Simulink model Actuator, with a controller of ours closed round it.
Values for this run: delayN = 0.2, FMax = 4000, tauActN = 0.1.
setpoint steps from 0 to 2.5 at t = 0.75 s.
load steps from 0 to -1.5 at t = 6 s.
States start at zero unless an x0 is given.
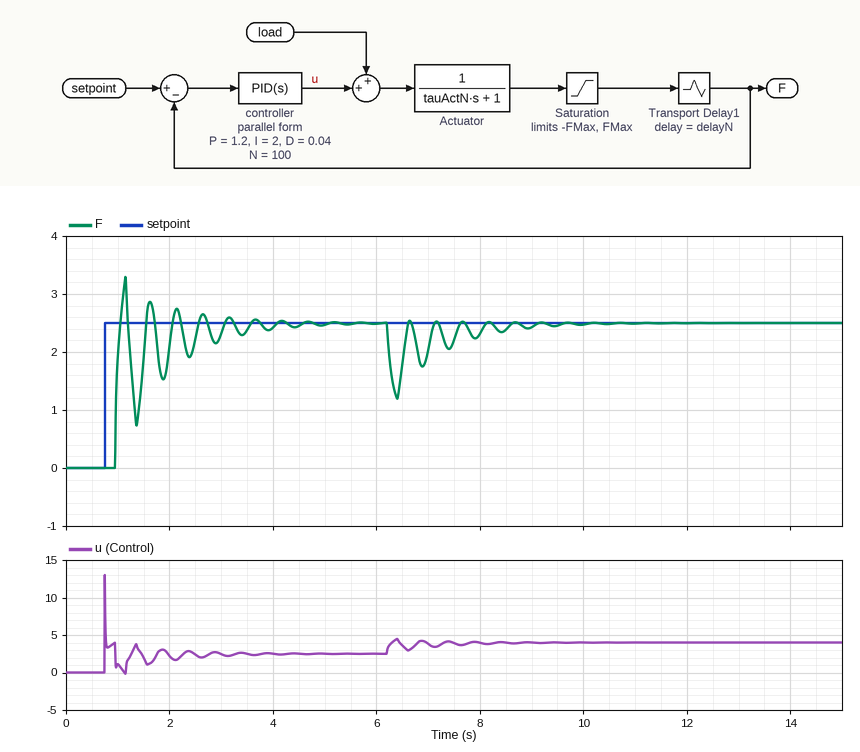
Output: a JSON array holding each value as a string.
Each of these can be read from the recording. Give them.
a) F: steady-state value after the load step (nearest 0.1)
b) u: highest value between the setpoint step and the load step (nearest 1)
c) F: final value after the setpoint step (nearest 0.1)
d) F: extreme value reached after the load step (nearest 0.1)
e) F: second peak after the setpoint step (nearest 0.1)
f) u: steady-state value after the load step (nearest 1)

["2.5", "13", "2.5", "1.2", "2.9", "4"]
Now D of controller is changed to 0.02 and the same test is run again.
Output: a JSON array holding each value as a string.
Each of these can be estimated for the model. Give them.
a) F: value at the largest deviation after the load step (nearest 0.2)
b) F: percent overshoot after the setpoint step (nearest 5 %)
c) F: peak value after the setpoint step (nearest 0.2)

["1.2", "30 %", "3.2"]
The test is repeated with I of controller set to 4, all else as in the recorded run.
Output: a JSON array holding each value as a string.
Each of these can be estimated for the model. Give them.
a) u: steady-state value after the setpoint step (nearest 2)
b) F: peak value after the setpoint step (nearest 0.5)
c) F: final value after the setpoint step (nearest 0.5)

["2", "4.0", "2.5"]
